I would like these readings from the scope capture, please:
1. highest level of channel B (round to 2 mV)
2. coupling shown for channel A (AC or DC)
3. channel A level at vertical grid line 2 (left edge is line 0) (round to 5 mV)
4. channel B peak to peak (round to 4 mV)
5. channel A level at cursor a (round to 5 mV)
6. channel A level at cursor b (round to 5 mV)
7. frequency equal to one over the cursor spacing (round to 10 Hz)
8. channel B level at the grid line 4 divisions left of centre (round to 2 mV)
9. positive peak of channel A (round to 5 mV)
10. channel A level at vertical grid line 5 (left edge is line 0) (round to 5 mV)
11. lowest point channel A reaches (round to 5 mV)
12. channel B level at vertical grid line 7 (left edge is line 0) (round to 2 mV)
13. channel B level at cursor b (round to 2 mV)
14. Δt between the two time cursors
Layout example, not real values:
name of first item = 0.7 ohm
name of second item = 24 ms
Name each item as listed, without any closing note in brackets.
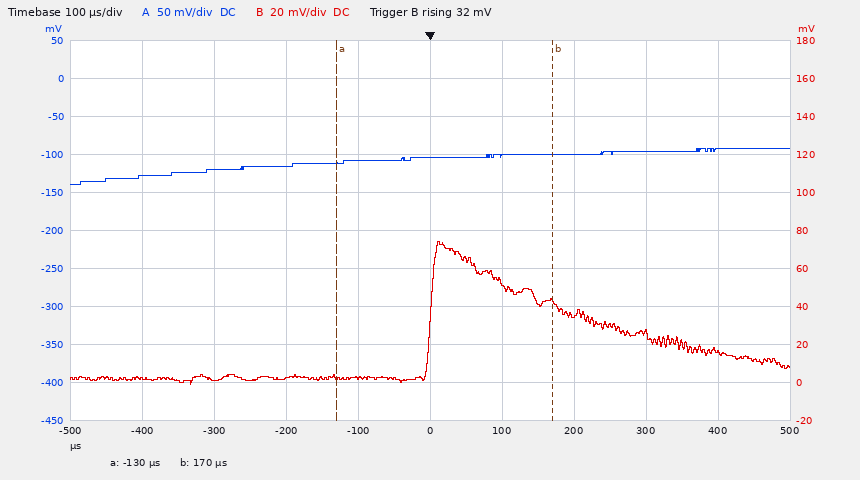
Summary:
highest level of channel B = 74 mV
coupling shown for channel A = DC
channel A level at vertical grid line 2 (left edge is line 0) = -120 mV
channel B peak to peak = 76 mV
channel A level at cursor a = -110 mV
channel A level at cursor b = -100 mV
frequency equal to one over the cursor spacing = 3.33 kHz
channel B level at the grid line 4 divisions left of centre = 2 mV
positive peak of channel A = -90 mV
channel A level at vertical grid line 5 (left edge is line 0) = -105 mV
lowest point channel A reaches = -140 mV
channel B level at vertical grid line 7 (left edge is line 0) = 36 mV
channel B level at cursor b = 42 mV
Δt between the two time cursors = 300 µs
